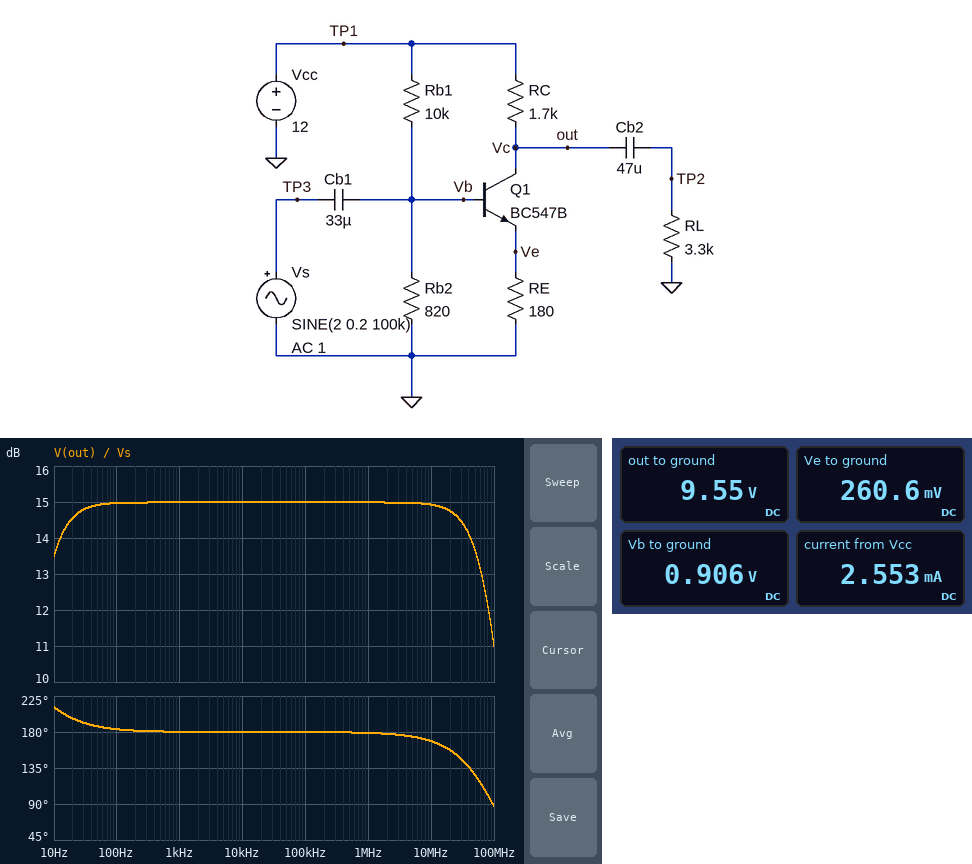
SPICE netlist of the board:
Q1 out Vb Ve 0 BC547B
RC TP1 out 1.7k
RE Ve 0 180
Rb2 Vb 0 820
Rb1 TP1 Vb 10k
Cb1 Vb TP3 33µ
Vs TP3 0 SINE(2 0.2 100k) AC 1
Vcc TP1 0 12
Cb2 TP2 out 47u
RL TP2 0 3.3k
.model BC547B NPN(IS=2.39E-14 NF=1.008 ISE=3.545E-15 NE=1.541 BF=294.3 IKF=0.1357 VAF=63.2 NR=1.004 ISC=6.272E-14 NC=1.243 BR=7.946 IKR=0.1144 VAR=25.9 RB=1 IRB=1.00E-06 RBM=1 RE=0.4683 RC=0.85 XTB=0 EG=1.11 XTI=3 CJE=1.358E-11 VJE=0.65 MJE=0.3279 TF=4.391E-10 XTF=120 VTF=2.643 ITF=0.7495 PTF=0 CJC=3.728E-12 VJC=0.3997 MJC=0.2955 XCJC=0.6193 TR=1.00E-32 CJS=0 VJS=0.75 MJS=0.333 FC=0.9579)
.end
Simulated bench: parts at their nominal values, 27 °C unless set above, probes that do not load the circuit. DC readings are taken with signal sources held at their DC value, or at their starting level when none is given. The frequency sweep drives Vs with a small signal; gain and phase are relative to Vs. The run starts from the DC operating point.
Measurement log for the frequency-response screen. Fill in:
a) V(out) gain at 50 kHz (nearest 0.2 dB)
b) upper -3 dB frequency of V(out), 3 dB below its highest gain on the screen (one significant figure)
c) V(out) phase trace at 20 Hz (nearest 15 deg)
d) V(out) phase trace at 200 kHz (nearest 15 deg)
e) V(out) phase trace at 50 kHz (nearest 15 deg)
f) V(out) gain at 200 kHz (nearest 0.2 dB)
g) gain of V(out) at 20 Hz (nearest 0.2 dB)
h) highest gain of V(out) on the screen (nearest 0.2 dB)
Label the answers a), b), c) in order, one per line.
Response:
a) 15.0 dB
b) 80 MHz
c) 195 deg
d) 180 deg
e) 180 deg
f) 15.0 dB
g) 14.6 dB
h) 15.0 dB
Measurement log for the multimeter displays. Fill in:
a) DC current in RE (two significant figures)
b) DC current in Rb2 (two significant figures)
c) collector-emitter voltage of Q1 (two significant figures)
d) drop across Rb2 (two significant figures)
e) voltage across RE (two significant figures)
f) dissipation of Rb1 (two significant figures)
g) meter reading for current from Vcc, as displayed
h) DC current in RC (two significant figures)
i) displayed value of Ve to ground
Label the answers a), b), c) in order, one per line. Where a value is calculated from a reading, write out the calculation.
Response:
a) (260.6 mV) / 180 Ω = 1.4 mA
b) (906 mV) / 820 Ω = 1.1 mA
c) 9.55 V - 260.6 mV = 9.3 V
d) 906 mV = 910 mV
e) 260.6 mV = 260 mV
f) (12 V - 906 mV)^2 / 10 kΩ = 12 mW
g) 2.553 mA
h) (12 V - 9.55 V) / 1.7 kΩ = 1.4 mA
i) 260.6 mV
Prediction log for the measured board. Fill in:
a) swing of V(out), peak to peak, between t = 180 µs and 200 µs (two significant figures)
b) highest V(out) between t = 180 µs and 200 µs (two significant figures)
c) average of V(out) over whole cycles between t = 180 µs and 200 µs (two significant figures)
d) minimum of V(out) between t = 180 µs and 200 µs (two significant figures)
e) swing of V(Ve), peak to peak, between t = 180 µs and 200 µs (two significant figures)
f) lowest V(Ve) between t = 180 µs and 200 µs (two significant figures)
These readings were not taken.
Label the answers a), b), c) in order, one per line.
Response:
a) 2.2 V
b) 11 V
c) 9.5 V
d) 8.4 V
e) 360 mV
f) 90 mV
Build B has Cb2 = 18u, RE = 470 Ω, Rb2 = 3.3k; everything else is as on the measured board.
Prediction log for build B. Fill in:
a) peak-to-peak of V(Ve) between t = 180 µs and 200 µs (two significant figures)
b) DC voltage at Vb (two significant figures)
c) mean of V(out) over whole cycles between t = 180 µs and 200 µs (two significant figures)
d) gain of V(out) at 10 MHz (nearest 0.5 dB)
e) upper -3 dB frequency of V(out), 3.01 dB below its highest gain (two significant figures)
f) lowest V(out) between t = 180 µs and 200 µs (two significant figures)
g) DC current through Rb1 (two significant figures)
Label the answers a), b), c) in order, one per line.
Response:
a) 390 mV
b) 2.9 V
c) 3.9 V
d) 7.5 dB
e) 87 MHz
f) 3.4 V
g) 910 µA
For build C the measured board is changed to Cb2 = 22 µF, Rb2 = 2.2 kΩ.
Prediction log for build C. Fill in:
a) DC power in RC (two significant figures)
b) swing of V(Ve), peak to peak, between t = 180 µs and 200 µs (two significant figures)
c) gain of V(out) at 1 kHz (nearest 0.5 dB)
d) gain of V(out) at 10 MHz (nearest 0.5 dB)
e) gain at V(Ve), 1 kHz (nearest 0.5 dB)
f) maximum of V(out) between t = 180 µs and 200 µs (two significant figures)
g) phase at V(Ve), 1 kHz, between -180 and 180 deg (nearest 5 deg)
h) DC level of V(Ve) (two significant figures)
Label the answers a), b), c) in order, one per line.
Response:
a) 68 mW
b) 370 mV
c) -21.5 dB
d) -4.5 dB
e) -1.5 dB
f) 2.3 V
g) 0 deg
h) 1.2 V
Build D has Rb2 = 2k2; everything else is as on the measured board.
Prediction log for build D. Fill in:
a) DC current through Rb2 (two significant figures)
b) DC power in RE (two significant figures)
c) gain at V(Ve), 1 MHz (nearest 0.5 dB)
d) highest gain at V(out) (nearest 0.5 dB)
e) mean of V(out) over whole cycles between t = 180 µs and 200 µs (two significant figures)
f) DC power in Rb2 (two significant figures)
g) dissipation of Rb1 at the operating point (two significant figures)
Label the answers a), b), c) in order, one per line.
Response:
a) 850 µA
b) 7.6 mW
c) -1.5 dB
d) 0 dB
e) 1.6 V
f) 1.6 mW
g) 10 mW
